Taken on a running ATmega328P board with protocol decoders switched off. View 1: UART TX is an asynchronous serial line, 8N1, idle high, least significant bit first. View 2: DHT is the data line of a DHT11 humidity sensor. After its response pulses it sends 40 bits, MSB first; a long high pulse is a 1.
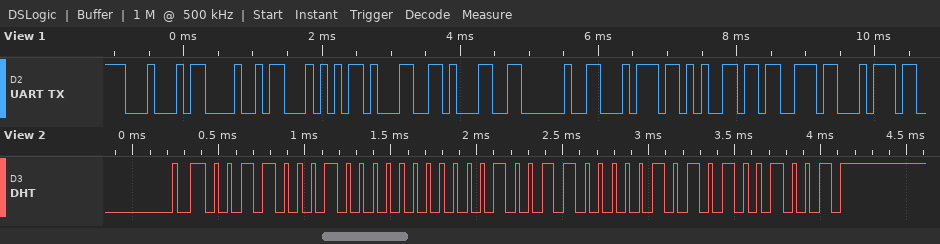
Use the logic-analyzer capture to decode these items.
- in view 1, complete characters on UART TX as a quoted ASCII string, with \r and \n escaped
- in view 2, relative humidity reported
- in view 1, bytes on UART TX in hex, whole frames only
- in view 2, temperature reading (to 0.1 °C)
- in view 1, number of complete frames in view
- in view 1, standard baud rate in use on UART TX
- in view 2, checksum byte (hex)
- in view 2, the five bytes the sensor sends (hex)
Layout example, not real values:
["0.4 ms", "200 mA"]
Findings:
["\"DHT11 test\"", "49 %", "44 48 54 31 31 20 74 65 73 74", "19.5 °C", "10", "9600 baud", "0x49", "31 00 13 05 49"]
